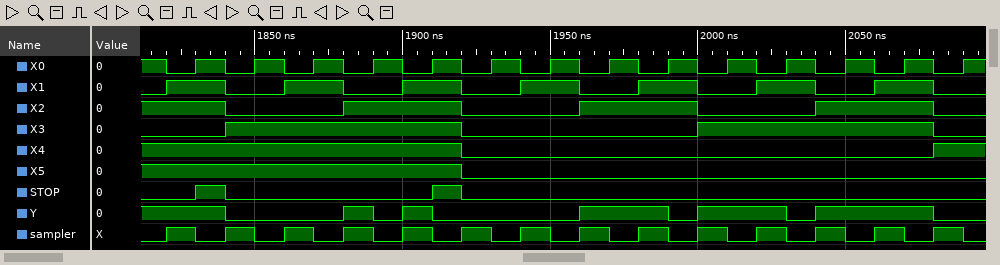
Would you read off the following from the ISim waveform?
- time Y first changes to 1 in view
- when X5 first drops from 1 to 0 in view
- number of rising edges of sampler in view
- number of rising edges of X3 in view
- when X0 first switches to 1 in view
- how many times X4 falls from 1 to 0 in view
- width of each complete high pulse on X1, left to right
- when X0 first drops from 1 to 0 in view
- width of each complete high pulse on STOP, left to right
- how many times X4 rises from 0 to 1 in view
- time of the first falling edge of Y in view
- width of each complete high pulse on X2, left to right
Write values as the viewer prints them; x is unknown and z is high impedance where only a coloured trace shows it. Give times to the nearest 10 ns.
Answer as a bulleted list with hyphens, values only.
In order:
- 1880 ns
- 1920 ns
- 14
- 2
- 1830 ns
- 1
- 20 ns, 20 ns, 20 ns, 20 ns, 20 ns, 20 ns, 20 ns
- 1820 ns
- 10 ns, 10 ns
- 1
- 1840 ns
- 40 ns, 40 ns, 40 ns
